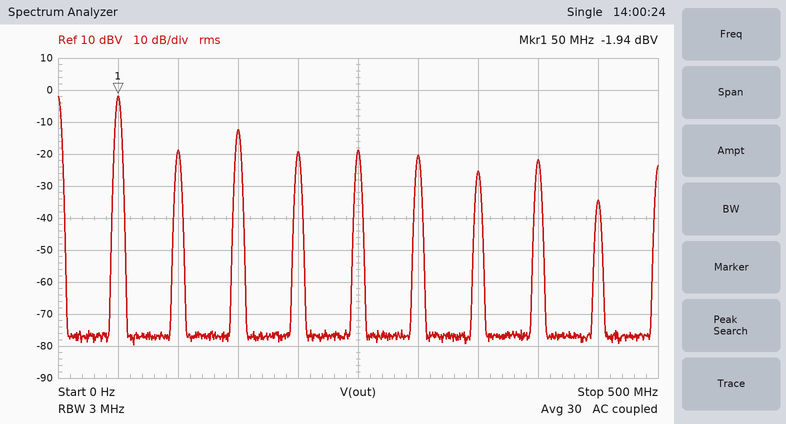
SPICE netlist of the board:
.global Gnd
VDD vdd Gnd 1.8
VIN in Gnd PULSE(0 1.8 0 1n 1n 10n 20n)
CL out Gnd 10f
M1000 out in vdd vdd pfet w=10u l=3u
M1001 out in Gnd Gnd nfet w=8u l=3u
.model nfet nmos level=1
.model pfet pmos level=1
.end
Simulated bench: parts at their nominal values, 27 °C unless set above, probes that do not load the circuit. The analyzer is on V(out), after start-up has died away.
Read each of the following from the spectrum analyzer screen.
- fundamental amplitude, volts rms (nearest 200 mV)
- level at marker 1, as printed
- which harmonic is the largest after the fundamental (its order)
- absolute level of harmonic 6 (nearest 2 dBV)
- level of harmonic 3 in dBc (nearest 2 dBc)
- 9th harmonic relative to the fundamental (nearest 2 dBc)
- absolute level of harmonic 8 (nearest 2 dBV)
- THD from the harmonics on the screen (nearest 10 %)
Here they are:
800 mV
-1.94 dBV
3
-20 dBV
-10 dBc
-32 dBc
-22 dBV
40 %
